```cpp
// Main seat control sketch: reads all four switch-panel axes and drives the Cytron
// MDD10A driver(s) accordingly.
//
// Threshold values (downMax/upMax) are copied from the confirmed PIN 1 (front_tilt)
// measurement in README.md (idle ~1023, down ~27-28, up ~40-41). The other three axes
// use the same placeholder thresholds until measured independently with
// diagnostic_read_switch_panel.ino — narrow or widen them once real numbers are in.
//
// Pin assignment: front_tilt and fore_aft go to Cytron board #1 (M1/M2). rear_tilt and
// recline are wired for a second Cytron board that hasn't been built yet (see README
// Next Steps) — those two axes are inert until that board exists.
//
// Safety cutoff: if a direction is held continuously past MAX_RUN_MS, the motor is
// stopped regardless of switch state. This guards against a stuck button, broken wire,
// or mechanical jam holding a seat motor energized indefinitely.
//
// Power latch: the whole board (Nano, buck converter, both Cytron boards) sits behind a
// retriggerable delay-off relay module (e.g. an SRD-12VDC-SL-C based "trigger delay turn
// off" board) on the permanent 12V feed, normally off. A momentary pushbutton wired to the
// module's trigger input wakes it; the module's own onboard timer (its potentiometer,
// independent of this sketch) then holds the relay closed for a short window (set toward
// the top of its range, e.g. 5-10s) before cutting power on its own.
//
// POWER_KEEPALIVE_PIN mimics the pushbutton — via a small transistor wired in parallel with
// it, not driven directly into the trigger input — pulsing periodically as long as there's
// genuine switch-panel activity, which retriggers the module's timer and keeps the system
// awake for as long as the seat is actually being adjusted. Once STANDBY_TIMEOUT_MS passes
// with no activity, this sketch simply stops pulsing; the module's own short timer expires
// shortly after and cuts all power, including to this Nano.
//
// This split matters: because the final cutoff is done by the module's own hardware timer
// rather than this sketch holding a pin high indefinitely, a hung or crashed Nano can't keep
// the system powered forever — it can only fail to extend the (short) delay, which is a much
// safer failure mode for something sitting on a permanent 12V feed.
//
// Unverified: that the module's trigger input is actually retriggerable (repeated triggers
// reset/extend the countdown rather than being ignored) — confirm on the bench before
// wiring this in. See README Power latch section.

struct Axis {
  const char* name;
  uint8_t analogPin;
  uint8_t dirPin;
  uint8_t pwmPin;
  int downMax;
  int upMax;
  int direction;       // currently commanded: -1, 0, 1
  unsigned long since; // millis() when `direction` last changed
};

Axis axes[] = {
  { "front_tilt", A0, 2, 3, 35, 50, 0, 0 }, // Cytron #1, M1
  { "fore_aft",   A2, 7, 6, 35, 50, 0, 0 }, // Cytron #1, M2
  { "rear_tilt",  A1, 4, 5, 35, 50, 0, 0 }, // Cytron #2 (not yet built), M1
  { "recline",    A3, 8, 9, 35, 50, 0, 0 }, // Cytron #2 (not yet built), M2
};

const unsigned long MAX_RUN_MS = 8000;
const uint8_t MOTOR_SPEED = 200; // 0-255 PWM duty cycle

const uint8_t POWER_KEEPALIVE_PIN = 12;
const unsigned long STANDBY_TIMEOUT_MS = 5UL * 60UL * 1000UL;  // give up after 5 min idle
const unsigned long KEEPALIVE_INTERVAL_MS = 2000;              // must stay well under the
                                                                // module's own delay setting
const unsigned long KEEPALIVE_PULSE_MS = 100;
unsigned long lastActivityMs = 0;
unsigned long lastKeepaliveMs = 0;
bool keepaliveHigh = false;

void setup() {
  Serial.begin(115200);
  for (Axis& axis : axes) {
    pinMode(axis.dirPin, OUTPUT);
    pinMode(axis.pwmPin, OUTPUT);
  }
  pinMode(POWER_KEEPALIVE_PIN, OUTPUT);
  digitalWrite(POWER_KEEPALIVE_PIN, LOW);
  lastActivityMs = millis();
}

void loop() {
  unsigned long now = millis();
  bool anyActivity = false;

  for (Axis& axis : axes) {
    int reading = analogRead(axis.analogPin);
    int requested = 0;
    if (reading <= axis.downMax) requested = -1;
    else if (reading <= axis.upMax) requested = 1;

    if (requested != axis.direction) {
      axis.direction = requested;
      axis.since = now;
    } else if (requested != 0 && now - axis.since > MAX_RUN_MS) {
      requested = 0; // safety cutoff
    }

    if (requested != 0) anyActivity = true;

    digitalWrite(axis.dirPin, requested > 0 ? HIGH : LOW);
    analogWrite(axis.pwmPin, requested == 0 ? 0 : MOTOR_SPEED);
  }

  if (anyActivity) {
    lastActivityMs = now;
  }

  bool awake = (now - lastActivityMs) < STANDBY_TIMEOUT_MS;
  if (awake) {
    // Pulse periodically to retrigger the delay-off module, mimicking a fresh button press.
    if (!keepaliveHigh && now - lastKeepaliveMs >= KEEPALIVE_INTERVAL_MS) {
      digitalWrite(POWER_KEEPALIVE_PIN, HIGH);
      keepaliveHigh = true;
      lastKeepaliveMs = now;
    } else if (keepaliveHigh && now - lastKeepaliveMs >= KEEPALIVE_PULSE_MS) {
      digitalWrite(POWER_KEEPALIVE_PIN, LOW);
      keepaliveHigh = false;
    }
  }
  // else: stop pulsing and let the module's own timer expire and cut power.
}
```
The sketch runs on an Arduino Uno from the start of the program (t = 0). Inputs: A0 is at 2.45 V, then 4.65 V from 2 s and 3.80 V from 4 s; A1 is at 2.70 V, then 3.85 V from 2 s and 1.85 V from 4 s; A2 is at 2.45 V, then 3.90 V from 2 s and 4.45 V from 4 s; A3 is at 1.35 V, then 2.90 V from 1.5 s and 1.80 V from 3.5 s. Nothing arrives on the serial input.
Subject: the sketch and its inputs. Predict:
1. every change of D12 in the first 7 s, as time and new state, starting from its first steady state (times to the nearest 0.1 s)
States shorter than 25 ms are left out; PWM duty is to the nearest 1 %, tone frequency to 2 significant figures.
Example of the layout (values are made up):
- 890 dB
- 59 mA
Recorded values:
- 0 s low; 2 s high; 2.1 s low; 4 s high; 4.1 s low; 6 s high; 6.1 s low
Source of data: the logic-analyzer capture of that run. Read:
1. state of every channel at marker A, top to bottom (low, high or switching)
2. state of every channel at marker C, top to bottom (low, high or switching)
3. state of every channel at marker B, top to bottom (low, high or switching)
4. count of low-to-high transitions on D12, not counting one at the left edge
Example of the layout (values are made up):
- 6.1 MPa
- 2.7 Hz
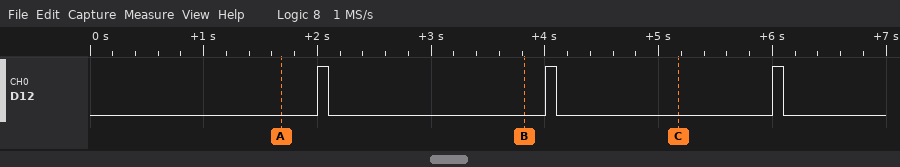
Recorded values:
- D12 low
- D12 low
- D12 low
- 3
